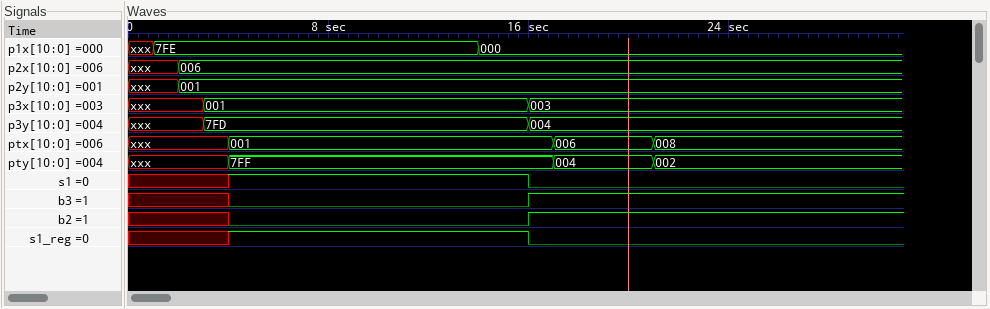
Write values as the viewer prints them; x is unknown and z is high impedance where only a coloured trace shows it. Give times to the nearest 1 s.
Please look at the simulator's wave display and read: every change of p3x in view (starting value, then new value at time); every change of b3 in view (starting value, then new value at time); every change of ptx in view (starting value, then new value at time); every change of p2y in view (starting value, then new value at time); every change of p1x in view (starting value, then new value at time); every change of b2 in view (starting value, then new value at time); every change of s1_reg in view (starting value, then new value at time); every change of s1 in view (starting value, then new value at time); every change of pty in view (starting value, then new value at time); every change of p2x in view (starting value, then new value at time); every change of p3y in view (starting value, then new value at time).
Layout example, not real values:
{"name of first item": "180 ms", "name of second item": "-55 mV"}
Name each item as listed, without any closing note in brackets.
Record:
{"every change of p3x in view": "xxx, 001 at 3 s, 003 at 16 s", "every change of b3 in view": "x, 0 at 4 s, 1 at 16 s", "every change of ptx in view": "xxx, 001 at 4 s, 006 at 17 s, 008 at 21 s", "every change of p2y in view": "xxx, 001 at 2 s", "every change of p1x in view": "xxx, 7FE at 1 s, 000 at 14 s", "every change of b2 in view": "x, 0 at 4 s, 1 at 16 s", "every change of s1_reg in view": "x, 1 at 4 s, 0 at 16 s", "every change of s1 in view": "x, 1 at 4 s, 0 at 16 s", "every change of pty in view": "xxx, 7FF at 4 s, 004 at 17 s, 002 at 21 s", "every change of p2x in view": "xxx, 006 at 2 s", "every change of p3y in view": "xxx, 7FD at 3 s, 004 at 16 s"}
